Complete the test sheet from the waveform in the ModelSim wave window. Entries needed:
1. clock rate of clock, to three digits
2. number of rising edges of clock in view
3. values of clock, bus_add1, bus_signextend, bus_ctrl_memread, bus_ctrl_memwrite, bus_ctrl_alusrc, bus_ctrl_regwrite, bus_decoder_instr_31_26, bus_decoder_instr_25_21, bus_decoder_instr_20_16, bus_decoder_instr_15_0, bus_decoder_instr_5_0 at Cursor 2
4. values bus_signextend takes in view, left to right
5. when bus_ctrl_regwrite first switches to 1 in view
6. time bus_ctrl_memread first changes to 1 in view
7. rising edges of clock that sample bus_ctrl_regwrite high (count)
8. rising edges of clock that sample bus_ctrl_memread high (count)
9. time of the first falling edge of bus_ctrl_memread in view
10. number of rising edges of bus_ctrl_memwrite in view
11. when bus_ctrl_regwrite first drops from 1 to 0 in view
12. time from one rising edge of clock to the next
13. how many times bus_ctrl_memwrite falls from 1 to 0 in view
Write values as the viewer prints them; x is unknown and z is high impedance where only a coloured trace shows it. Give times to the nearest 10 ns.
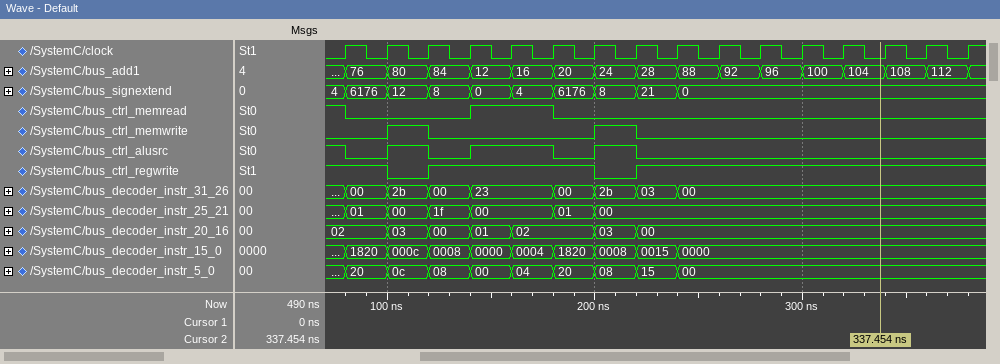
50.0 MHz
16
clock=0, bus_add1=104, bus_signextend=0, bus_ctrl_memread=0, bus_ctrl_memwrite=0, bus_ctrl_alusrc=0, bus_ctrl_regwrite=1, bus_decoder_instr_31_26=00, bus_decoder_instr_25_21=00, bus_decoder_instr_20_16=00, bus_decoder_instr_15_0=0000, bus_decoder_instr_5_0=00
4, 6176, 12, 8, 0, 4, 6176, 8, 21, 0
120 ns
140 ns
14
3
80 ns
2
100 ns
20 ns
2
